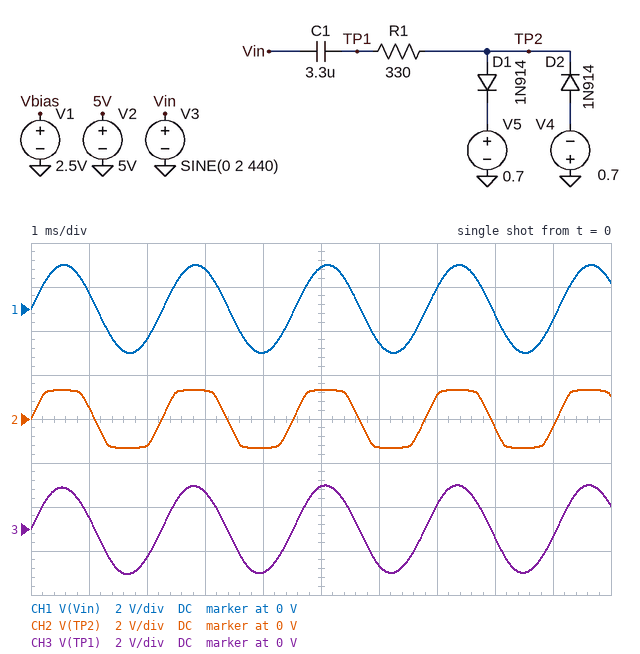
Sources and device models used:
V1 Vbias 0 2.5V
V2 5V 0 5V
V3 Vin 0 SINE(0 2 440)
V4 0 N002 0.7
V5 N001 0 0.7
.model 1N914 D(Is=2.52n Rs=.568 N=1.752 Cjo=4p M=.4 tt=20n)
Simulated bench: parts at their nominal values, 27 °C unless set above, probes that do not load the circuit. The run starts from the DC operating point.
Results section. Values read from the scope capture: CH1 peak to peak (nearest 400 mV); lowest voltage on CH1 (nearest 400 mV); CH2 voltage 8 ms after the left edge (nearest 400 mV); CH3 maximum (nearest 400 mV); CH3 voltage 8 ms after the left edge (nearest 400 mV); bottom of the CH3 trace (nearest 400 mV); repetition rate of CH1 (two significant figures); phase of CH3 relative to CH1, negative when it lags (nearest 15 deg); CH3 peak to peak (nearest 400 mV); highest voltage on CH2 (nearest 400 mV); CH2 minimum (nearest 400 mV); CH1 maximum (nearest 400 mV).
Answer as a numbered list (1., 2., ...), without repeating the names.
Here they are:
1. 4.0 V
2. -2.0 V
3. -400 mV
4. 2.0 V
5. -400 mV
6. -2.0 V
7. 440 Hz
8. 0 deg
9. 4.0 V
10. 1.2 V
11. -1.2 V
12. 2.0 V
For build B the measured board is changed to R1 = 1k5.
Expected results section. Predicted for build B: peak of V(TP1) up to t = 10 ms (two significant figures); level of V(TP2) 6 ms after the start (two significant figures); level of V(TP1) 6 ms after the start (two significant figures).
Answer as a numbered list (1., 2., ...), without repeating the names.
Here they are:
1. 2.0 V
2. -1.2 V
3. -1.6 V
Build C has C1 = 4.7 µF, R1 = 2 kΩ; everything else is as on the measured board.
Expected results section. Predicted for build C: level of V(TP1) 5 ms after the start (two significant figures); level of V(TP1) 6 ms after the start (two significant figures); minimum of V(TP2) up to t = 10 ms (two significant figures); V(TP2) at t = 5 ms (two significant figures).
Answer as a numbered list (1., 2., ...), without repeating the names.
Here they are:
1. 1.9 V
2. -1.6 V
3. -1.2 V
4. 1.2 V
